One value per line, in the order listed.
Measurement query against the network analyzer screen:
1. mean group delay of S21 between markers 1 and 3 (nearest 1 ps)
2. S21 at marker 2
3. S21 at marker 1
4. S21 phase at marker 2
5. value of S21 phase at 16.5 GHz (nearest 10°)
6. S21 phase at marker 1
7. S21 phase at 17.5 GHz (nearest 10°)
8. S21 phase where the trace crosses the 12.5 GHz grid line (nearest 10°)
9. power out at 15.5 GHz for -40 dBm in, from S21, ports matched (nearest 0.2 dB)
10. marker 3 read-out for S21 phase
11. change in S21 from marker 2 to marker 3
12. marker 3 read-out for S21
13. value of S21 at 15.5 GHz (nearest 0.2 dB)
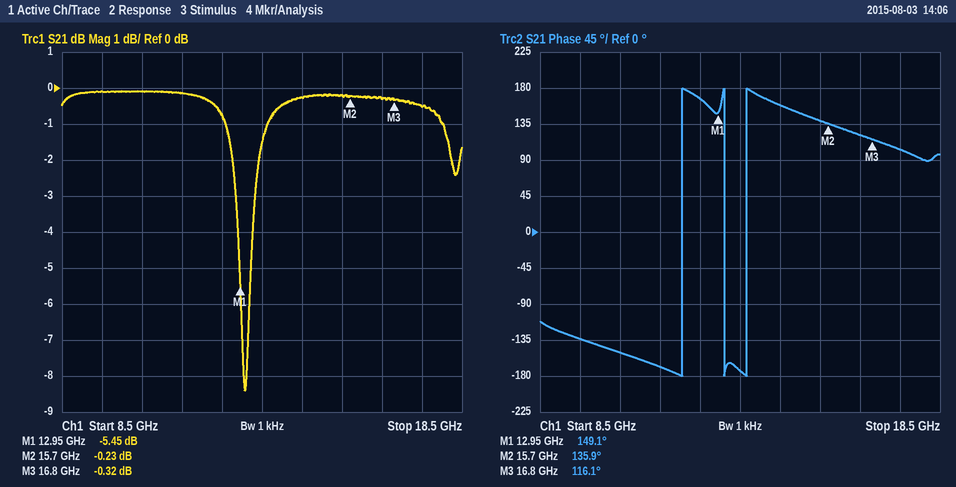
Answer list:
24 ps
-0.23 dB
-5.45 dB
135.9°
120°
149.1°
100°
170°
-40.2 dBm
116.1°
-0.09 dB
-0.32 dB
-0.2 dB
